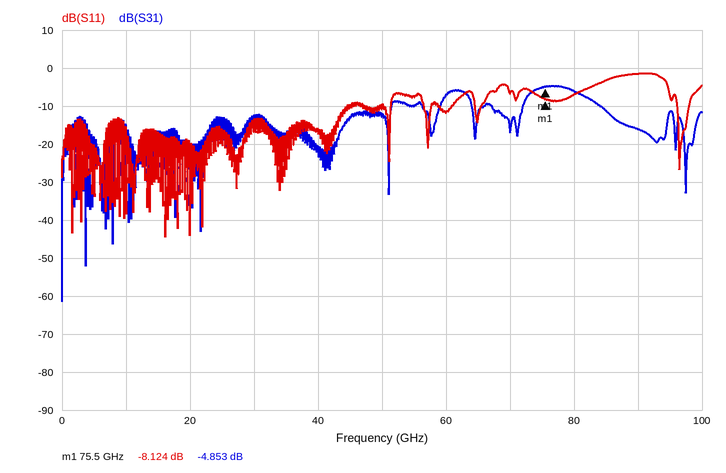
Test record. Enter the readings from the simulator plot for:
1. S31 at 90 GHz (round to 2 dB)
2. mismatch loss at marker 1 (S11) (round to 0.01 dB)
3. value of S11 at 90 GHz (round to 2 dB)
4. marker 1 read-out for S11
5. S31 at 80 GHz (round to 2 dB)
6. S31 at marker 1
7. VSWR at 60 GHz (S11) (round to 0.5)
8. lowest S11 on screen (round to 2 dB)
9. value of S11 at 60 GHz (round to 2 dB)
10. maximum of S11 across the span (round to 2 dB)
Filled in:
-16 dB
0.73 dB
-2 dB
-8.124 dB
-6 dB
-4.853 dB
1.5
-44 dB
-12 dB
-2 dB
